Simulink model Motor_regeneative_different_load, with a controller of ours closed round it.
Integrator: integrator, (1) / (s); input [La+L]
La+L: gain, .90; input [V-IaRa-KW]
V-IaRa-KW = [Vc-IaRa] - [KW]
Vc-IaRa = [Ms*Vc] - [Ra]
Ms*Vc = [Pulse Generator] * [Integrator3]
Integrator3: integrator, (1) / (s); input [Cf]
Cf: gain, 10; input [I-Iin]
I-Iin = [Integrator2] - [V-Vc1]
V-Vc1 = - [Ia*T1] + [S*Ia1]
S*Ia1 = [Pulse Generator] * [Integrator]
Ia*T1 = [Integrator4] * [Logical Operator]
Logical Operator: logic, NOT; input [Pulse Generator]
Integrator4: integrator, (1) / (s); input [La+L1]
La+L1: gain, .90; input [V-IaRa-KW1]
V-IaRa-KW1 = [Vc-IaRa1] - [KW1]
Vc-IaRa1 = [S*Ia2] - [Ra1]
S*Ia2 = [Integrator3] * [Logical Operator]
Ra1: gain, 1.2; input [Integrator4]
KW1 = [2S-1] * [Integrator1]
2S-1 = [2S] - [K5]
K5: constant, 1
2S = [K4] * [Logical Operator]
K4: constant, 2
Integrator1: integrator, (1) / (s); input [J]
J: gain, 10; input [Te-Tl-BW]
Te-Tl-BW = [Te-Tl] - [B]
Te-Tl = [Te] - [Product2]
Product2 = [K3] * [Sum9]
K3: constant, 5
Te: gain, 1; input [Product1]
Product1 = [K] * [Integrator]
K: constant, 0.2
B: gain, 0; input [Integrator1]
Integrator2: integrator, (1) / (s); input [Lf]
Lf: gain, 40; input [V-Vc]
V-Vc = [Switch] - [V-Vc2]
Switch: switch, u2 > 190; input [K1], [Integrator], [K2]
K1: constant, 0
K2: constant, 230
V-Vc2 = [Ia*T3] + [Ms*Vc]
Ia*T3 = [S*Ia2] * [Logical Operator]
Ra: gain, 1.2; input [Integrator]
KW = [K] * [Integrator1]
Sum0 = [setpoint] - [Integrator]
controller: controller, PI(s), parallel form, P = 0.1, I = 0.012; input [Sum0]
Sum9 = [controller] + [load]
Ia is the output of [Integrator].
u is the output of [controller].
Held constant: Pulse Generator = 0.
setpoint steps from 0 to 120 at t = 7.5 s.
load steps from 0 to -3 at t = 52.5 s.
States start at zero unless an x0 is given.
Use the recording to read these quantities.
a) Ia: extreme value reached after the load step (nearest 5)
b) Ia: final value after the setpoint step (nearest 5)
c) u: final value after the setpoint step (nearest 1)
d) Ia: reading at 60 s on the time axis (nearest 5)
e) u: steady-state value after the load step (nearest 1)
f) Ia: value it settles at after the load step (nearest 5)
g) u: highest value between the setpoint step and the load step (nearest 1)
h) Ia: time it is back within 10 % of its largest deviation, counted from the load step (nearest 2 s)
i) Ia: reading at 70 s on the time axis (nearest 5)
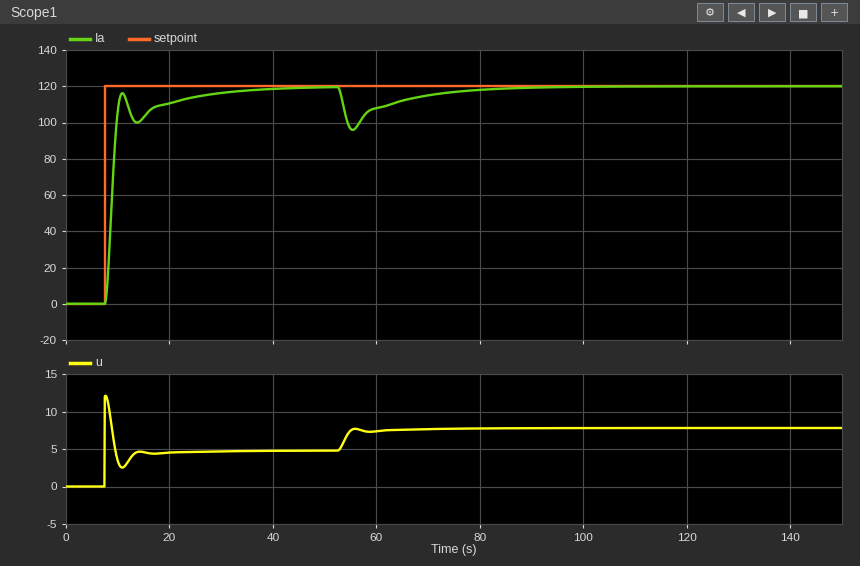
95
120
5
110
8
120
12
26 s
115
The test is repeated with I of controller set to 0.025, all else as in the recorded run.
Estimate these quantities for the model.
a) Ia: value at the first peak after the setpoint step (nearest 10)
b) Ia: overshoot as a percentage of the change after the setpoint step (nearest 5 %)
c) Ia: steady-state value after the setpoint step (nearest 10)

130
10 %
120
